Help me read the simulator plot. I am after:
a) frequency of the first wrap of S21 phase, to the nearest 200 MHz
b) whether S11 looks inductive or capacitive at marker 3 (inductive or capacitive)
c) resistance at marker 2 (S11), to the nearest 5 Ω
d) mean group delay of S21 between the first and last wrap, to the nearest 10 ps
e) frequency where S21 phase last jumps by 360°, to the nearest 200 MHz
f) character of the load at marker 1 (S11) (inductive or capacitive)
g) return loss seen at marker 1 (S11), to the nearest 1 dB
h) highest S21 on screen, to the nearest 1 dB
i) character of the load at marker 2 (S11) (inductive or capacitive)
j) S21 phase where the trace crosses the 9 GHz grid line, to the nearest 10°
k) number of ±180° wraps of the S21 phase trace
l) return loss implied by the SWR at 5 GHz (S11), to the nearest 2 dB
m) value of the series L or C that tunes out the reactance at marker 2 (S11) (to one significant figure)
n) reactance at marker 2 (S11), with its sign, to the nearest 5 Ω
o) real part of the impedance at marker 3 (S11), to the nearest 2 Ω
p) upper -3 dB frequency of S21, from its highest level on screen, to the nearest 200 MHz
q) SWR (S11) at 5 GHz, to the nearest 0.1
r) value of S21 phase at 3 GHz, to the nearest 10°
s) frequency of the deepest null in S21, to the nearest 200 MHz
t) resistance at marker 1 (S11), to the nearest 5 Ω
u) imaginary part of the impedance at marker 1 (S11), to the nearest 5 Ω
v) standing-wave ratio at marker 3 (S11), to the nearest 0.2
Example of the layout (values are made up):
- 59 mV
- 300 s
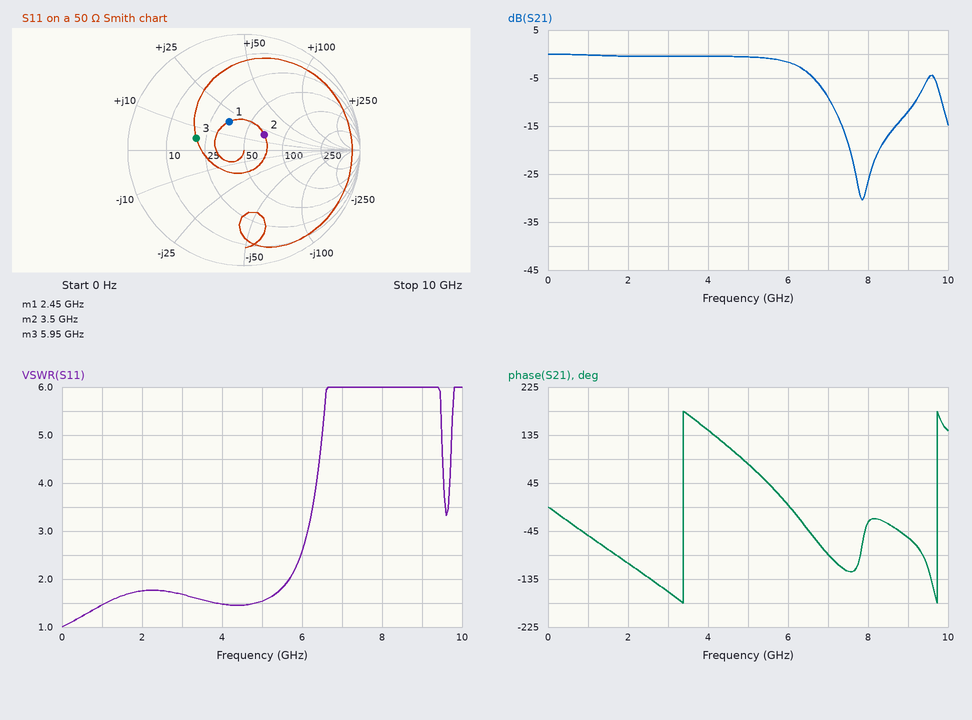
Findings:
- 3.4 GHz
- inductive
- 70 Ω
- 160 ps
- 9.8 GHz
- inductive
- 11 dB
- 0 dB
- inductive
- -60°
- 2
- 14 dB
- 2 pF
- +20 Ω
- 20 Ω
- 6.4 GHz
- 1.5
- -160°
- 7.8 GHz
- 35 Ω
- +20 Ω
- 2.4
